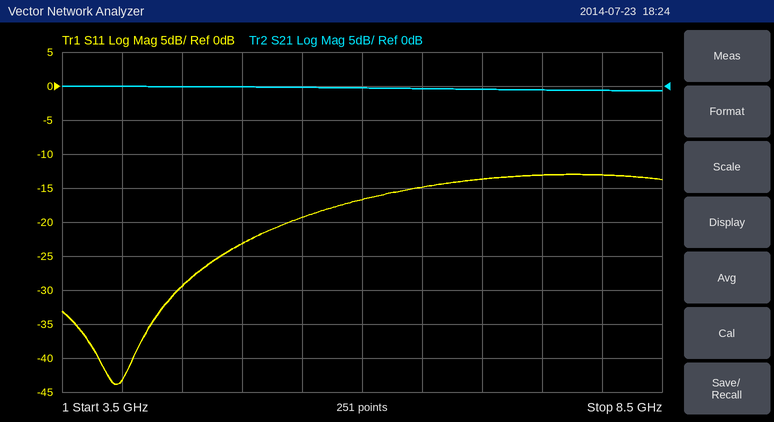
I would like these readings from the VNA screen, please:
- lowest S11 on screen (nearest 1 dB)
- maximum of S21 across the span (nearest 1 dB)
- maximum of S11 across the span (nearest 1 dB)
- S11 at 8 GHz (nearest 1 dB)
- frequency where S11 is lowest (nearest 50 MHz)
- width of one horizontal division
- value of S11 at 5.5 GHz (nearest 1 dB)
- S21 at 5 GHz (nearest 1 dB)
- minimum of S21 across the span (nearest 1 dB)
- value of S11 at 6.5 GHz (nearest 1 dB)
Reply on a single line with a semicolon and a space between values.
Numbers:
-44 dB; 0 dB; -13 dB; -13 dB; 3.95 GHz; 500 MHz; -19 dB; 0 dB; -1 dB; -15 dB
